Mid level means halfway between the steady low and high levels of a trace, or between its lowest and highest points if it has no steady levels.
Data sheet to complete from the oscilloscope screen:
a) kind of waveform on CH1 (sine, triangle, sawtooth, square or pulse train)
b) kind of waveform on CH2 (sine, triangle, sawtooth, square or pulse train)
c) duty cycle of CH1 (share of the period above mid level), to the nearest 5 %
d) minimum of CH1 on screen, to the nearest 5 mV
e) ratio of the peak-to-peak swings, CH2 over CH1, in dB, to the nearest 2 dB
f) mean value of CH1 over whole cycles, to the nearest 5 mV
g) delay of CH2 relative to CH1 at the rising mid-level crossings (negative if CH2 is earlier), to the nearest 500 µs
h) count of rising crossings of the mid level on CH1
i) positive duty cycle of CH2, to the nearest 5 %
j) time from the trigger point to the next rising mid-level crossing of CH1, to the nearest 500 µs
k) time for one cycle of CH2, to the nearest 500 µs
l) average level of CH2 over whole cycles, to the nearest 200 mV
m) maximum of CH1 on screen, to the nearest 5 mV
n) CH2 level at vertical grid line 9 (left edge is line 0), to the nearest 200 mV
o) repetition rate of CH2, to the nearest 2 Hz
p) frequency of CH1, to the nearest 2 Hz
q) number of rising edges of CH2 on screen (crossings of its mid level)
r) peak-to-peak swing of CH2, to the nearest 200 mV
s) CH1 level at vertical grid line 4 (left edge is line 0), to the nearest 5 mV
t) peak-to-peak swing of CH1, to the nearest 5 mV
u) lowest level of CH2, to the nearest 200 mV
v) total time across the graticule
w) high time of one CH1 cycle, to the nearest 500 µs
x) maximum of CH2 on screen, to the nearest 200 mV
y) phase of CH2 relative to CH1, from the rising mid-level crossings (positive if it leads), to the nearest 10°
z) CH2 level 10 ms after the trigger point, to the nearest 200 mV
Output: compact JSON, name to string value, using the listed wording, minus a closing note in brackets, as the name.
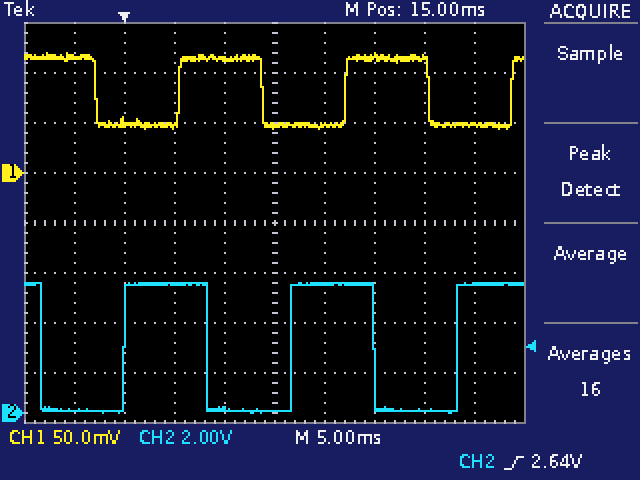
{"kind of waveform on CH1": "square", "kind of waveform on CH2": "square", "duty cycle of CH1 (share of the period above mid level), to the nearest 5 %": "50 %", "minimum of CH1 on screen, to the nearest 5 mV": "45 mV", "ratio of the peak-to-peak swings, CH2 over CH1, in dB, to the nearest 2 dB": "36 dB", "mean value of CH1 over whole cycles, to the nearest 5 mV": "80 mV", "delay of CH2 relative to CH1 at the rising mid-level crossings (negative if CH2 is earlier), to the nearest 500 µs": "-5.5 ms", "count of rising crossings of the mid level on CH1": "3", "positive duty cycle of CH2, to the nearest 5 %": "50 %", "time from the trigger point to the next rising mid-level crossing of CH1, to the nearest 500 µs": "5.5 ms", "time for one cycle of CH2, to the nearest 500 µs": "16.5 ms", "average level of CH2 over whole cycles, to the nearest 200 mV": "2.6 V", "maximum of CH1 on screen, to the nearest 5 mV": "120 mV", "CH2 level at vertical grid line 9 (left edge is line 0), to the nearest 200 mV": "5.2 V", "repetition rate of CH2, to the nearest 2 Hz": "60 Hz", "frequency of CH1, to the nearest 2 Hz": "60 Hz", "number of rising edges of CH2 on screen": "3", "peak-to-peak swing of CH2, to the nearest 200 mV": "5.2 V", "CH1 level at vertical grid line 4 (left edge is line 0), to the nearest 5 mV": "115 mV", "peak-to-peak swing of CH1, to the nearest 5 mV": "75 mV", "lowest level of CH2, to the nearest 200 mV": "0.0 V", "total time across the graticule": "50 ms", "high time of one CH1 cycle, to the nearest 500 µs": "8.5 ms", "maximum of CH2 on screen, to the nearest 200 mV": "5.2 V", "phase of CH2 relative to CH1, from the rising mid-level crossings (positive if it leads), to the nearest 10°": "+120°", "CH2 level 10 ms after the trigger point, to the nearest 200 mV": "200 mV"}
